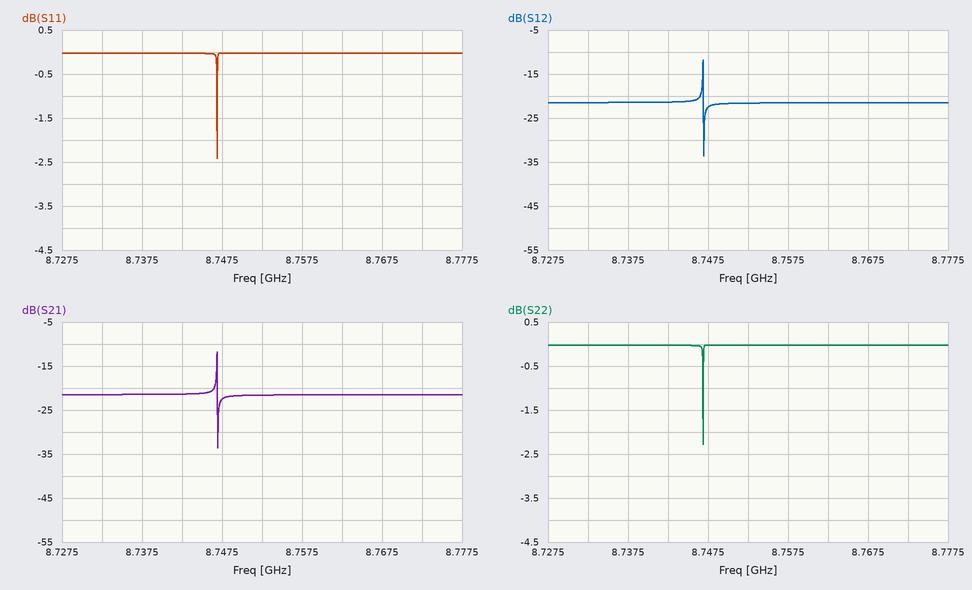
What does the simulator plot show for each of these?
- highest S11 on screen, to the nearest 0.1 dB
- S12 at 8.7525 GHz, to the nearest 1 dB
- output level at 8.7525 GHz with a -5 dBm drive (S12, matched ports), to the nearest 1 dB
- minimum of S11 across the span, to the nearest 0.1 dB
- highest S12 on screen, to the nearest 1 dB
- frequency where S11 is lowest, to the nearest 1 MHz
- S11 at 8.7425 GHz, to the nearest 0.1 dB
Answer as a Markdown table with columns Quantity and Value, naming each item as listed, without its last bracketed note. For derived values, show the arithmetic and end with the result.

| Quantity | Value |
|---|---|
| highest S11 on screen, to the nearest 0.1 dB | 0.0 dB |
| S12 at 8.7525 GHz, to the nearest 1 dB | -22 dB |
| output level at 8.7525 GHz with a -5 dBm drive (S12, matched ports), to the nearest 1 dB | -5 dBm + (-22 dB) = -27 dBm |
| minimum of S11 across the span, to the nearest 0.1 dB | -2.4 dB |
| highest S12 on screen, to the nearest 1 dB | -12 dB |
| frequency where S11 is lowest, to the nearest 1 MHz | 8.747 GHz |
| S11 at 8.7425 GHz, to the nearest 0.1 dB | 0.0 dB |
